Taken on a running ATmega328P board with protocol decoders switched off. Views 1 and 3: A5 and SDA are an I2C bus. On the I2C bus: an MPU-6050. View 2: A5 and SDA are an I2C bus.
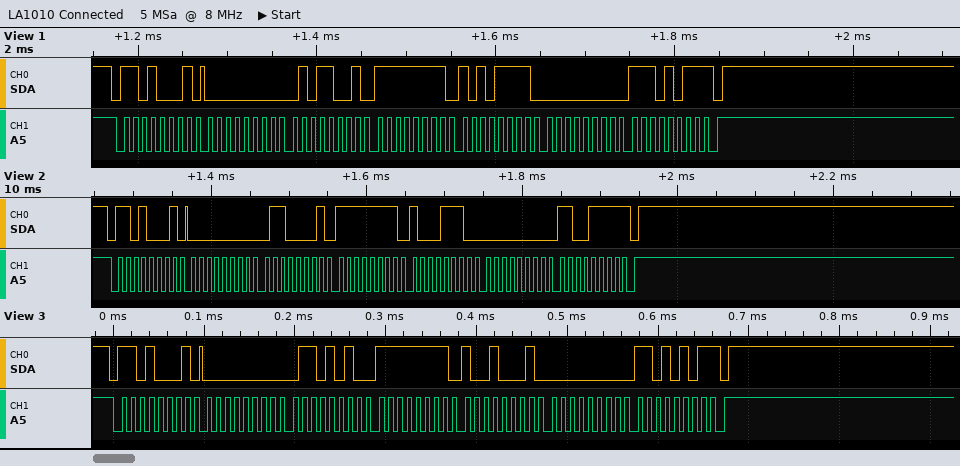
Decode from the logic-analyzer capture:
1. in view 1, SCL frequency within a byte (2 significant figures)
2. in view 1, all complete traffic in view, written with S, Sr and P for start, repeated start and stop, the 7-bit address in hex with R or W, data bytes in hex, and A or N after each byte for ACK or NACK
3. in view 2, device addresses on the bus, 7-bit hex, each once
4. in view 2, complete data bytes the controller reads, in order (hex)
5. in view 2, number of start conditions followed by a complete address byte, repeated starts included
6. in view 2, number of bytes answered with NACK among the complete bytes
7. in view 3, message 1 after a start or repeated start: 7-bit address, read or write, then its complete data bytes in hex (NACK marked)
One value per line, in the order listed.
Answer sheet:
100 kHz
S 68R A 00 A 59 A FF A AF A 00 A EB N P
0x68
00 61 FF 8E 00 CF
1
1
0x68 read: 00 6A FF 91 00 D5 NACK
